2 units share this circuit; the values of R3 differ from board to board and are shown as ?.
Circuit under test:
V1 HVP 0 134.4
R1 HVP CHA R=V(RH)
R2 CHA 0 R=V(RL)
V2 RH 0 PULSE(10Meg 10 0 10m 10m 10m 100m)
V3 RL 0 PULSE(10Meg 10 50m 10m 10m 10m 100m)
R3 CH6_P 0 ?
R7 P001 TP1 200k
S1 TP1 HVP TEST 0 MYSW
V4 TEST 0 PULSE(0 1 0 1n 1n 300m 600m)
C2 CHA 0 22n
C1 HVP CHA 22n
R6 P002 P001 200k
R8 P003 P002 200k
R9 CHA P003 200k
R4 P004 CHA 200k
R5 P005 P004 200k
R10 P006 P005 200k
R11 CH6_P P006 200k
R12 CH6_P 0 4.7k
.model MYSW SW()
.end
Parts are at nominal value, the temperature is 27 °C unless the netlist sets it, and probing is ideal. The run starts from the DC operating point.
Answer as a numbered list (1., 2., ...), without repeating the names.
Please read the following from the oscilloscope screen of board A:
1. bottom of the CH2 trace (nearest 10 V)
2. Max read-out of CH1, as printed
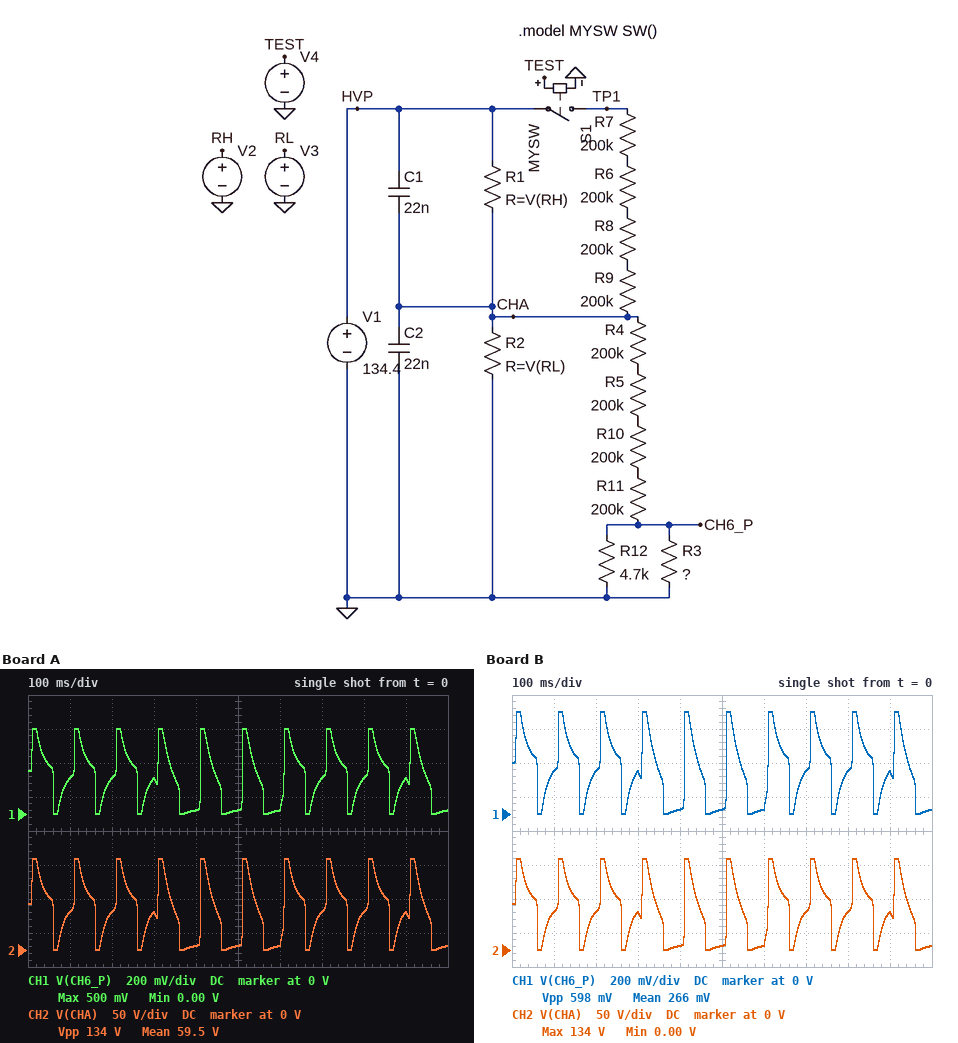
1. 0 V
2. 500 mV
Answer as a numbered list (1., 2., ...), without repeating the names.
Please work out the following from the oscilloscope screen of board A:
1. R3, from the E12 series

1. 8.2 kΩ
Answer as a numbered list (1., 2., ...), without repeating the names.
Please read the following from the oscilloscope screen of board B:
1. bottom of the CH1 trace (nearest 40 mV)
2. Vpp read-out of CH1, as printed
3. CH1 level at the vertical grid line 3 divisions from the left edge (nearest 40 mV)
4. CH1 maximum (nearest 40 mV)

1. 0 V
2. 598 mV
3. 240 mV
4. 600 mV
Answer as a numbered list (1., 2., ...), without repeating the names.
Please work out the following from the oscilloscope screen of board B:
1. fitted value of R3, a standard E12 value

1. 15 kΩ
